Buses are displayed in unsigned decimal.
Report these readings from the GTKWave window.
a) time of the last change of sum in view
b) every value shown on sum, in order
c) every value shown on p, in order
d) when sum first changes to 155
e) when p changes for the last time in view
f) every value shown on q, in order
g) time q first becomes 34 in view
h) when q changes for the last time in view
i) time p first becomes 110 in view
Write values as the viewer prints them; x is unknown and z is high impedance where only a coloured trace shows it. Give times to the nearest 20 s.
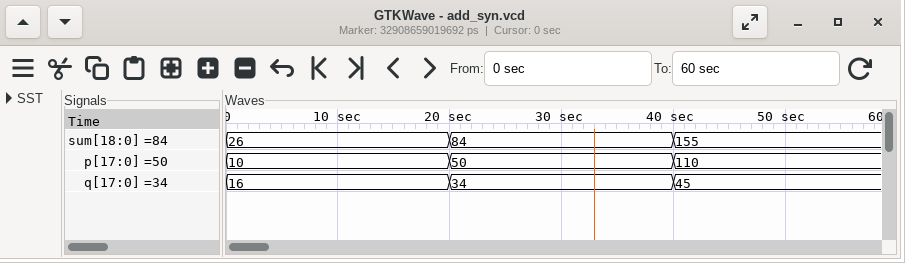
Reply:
40 s
26, 84, 155
10, 50, 110
40 s
40 s
16, 34, 45
20 s
40 s
40 s
